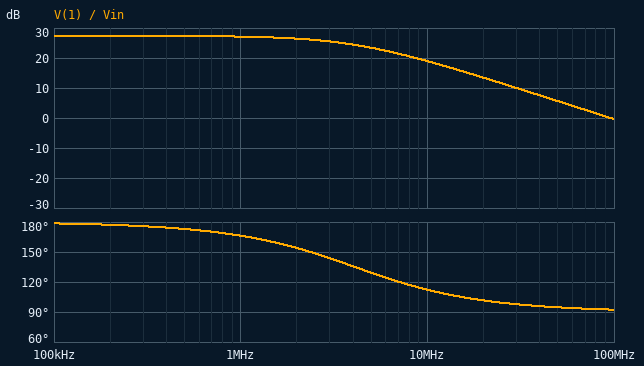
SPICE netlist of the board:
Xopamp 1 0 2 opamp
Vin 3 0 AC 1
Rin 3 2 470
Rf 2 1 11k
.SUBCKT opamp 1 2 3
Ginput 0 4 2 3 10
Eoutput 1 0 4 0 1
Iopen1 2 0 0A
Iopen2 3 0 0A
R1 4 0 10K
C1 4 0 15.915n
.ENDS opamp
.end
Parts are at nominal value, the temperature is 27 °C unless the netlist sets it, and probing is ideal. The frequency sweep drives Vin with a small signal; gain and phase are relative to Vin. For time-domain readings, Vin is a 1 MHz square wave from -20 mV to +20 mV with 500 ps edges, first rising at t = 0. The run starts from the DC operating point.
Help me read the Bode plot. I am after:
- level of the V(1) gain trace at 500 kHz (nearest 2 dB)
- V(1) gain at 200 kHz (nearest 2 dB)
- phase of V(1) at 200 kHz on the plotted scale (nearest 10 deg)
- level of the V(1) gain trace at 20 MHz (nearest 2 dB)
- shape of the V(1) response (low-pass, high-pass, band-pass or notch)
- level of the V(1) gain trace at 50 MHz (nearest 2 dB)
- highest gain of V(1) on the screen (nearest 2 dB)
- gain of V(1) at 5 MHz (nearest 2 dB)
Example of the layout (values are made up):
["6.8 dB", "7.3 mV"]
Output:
["28 dB", "28 dB", "180 deg", "14 dB", "low-pass", "6 dB", "28 dB", "24 dB"]
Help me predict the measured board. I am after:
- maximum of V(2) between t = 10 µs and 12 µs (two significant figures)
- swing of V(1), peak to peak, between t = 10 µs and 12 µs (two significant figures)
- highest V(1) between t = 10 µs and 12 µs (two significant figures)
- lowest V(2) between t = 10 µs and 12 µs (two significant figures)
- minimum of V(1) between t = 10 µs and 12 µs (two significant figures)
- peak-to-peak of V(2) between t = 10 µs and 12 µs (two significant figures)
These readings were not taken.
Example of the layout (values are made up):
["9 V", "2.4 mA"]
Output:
["38 mV", "940 mV", "470 mV", "-38 mV", "-470 mV", "76 mV"]
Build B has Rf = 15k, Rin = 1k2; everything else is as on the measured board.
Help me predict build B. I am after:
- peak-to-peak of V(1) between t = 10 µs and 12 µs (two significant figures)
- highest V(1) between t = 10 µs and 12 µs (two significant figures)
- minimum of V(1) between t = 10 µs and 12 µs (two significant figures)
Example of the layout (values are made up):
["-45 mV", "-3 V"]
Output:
["500 mV", "250 mV", "-250 mV"]
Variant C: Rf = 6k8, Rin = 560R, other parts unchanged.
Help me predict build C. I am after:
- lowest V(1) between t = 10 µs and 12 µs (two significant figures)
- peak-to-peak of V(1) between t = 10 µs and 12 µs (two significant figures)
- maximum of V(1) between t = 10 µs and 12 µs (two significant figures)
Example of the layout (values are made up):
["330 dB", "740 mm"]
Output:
["-240 mV", "490 mV", "240 mV"]
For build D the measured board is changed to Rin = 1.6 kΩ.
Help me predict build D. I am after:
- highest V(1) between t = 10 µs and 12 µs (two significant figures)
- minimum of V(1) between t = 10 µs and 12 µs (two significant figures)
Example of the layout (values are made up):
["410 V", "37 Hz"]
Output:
["140 mV", "-140 mV"]
